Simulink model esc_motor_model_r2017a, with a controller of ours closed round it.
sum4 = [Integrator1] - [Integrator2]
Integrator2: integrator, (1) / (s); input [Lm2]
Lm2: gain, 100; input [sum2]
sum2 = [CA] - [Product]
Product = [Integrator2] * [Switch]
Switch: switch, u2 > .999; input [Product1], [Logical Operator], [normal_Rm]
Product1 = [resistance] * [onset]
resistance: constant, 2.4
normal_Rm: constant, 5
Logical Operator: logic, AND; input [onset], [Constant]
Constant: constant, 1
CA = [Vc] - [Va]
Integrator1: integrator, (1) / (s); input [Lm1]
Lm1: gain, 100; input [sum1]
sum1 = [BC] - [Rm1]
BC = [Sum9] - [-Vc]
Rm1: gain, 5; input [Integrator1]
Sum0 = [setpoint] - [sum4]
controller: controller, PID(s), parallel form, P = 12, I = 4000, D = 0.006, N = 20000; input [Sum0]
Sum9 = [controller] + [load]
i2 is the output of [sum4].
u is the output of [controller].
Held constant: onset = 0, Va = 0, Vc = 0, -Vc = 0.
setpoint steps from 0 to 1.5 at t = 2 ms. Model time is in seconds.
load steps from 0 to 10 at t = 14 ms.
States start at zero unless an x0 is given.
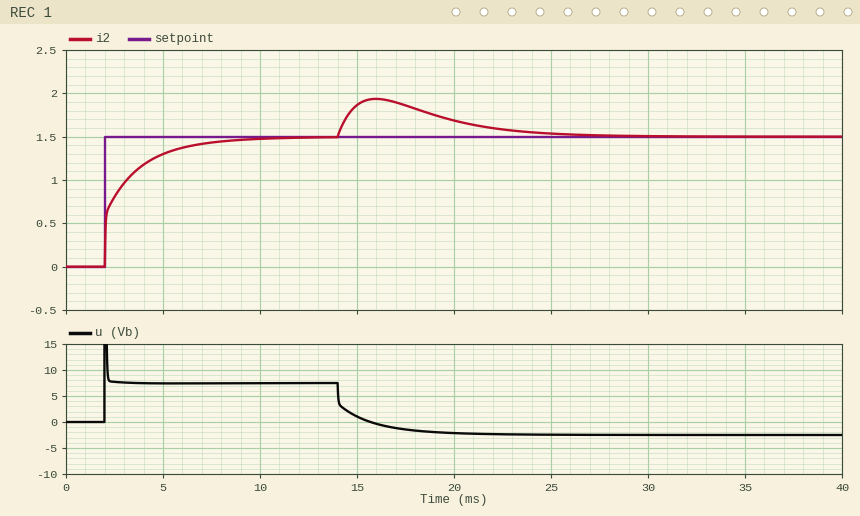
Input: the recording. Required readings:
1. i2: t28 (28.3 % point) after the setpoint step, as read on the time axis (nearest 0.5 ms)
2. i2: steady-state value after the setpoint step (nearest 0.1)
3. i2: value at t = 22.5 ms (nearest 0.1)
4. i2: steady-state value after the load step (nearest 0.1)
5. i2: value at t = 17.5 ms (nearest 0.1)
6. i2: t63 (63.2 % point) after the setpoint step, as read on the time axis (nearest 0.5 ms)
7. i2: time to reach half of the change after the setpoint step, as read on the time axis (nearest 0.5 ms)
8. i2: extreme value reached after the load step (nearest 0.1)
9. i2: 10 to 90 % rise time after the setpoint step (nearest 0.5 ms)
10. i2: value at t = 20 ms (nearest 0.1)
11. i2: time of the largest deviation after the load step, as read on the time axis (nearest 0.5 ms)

2.0 ms
1.5
1.6
1.5
1.9
3.0 ms
2.5 ms
1.9
3.5 ms
1.7
16.0 ms
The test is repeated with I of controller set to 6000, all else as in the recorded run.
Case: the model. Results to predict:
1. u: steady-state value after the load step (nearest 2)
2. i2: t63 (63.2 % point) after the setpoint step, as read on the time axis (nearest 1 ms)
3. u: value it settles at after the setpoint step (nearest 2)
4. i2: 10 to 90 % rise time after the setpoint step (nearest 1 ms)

-2
3 ms
8
3 ms
